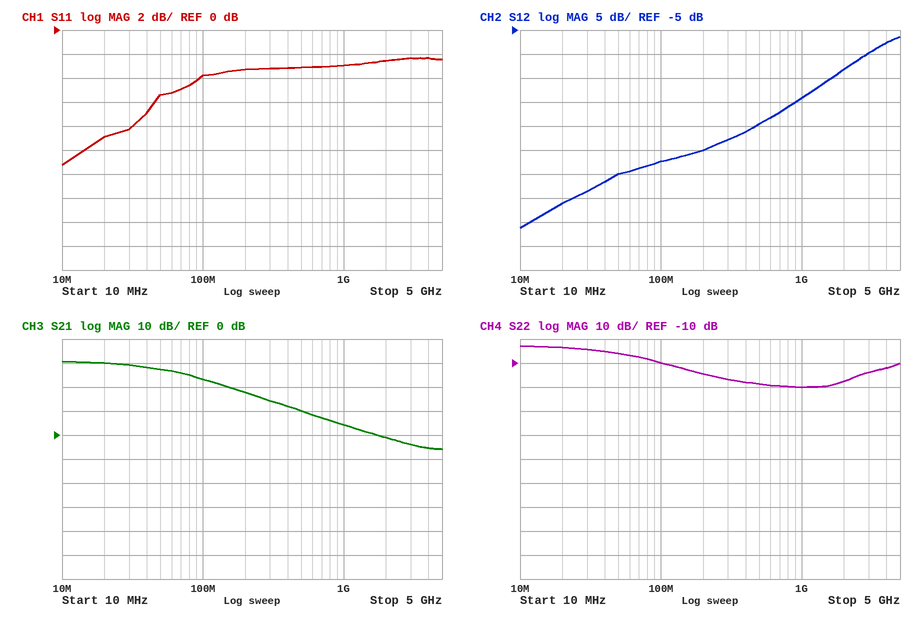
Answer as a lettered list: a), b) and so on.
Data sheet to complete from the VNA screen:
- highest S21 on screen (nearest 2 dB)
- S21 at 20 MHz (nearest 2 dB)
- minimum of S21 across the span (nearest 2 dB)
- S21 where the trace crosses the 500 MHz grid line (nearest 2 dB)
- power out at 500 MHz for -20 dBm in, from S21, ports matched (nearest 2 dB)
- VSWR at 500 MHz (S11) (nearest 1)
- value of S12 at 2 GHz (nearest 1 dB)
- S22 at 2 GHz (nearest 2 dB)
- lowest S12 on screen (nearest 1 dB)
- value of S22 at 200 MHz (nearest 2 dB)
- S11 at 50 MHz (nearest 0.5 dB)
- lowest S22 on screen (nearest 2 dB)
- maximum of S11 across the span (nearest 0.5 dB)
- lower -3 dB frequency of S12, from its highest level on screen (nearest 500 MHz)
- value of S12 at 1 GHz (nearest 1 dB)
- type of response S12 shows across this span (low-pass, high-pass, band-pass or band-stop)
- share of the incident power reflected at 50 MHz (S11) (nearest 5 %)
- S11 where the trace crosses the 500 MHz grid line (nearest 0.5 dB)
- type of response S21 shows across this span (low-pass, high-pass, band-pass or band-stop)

a) 30 dB
b) 30 dB
c) -6 dB
d) 10 dB
e) -10 dBm
f) 6
g) -13 dB
h) -18 dB
i) -46 dB
j) -14 dB
k) -5.5 dB
l) -20 dB
m) -2.5 dB
n) 3.0 GHz
o) -19 dB
p) high-pass
q) 30 %
r) -3.0 dB
s) low-pass
